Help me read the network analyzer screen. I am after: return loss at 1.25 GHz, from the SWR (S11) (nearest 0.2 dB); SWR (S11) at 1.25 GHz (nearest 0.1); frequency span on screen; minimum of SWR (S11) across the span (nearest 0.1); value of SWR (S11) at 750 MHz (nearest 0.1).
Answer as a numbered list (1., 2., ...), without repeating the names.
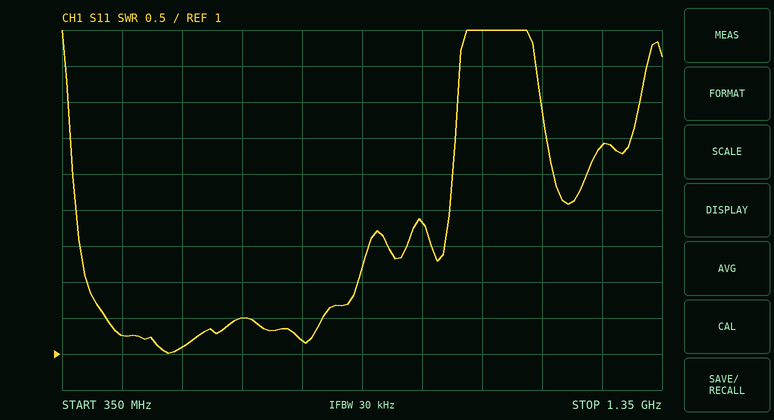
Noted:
1. 4.6 dB
2. 3.9
3. 1 GHz
4. 1.0
5. 1.2
